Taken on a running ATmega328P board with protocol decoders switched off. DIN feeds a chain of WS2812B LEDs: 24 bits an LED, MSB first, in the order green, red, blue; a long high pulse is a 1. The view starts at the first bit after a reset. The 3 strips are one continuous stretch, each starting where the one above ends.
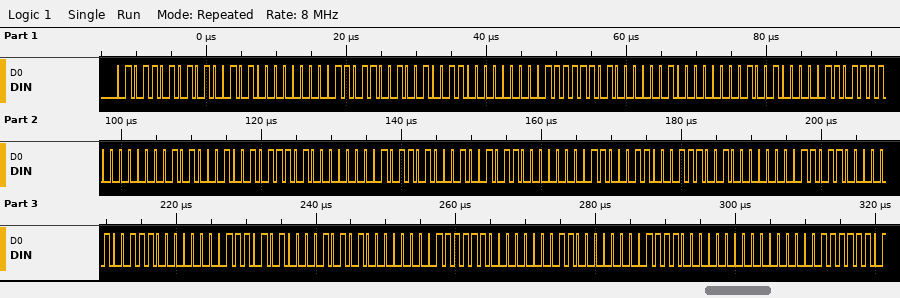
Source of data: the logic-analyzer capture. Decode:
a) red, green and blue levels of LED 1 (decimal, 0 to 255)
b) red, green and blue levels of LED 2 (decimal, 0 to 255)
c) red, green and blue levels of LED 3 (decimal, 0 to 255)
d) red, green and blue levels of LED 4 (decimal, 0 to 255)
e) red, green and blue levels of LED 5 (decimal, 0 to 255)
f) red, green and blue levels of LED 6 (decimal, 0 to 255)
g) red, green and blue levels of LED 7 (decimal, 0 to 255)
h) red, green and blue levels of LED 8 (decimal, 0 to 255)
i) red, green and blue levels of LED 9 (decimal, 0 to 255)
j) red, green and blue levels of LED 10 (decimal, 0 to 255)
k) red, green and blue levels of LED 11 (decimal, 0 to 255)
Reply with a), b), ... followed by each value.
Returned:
a) 165, 90, 0
b) 147, 108, 0
c) 129, 126, 0
d) 111, 144, 0
e) 93, 162, 0
f) 75, 180, 0
g) 57, 198, 0
h) 39, 216, 0
i) 21, 234, 0
j) 3, 252, 0
k) 0, 240, 15
